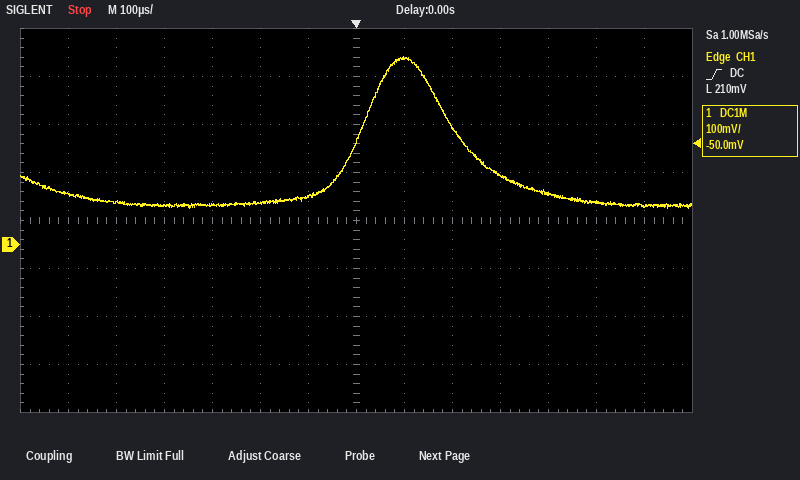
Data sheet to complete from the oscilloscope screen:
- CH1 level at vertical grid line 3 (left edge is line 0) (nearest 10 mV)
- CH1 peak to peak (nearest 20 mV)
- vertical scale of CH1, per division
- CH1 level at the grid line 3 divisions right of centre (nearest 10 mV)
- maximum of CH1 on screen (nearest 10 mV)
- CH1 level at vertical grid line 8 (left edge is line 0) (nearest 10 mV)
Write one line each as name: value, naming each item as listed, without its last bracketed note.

CH1 level at vertical grid line 3 (left edge is line 0): 80 mV
CH1 peak to peak: 320 mV
vertical scale of CH1, per division: 100 mV
CH1 level at the grid line 3 divisions right of centre: 140 mV
maximum of CH1 on screen: 390 mV
CH1 level at vertical grid line 8 (left edge is line 0): 390 mV
